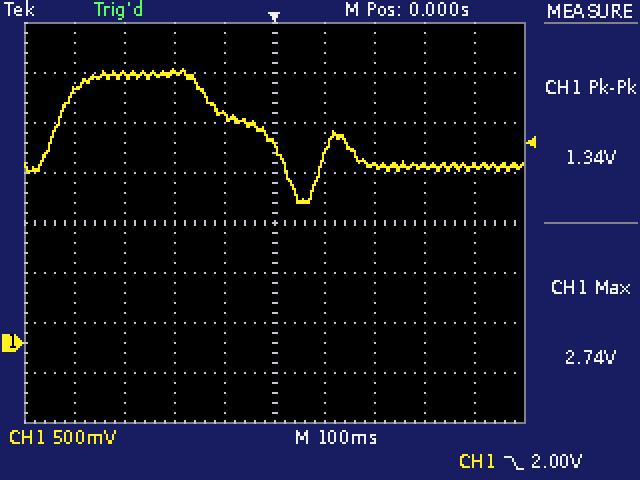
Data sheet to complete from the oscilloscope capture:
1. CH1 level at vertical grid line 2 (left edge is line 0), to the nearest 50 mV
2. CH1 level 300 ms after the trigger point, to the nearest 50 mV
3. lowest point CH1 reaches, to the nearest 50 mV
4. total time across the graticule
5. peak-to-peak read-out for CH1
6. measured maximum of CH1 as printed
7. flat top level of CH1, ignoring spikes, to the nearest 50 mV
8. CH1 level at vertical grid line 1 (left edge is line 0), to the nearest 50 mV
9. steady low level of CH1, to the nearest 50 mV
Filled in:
2.70 V
1.75 V
1.40 V
1 s
1.34 V
2.74 V
2.70 V
2.50 V
1.75 V
